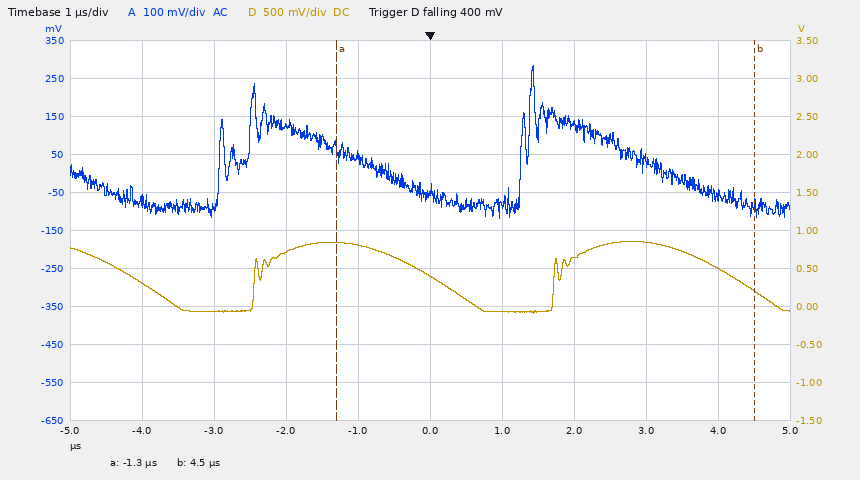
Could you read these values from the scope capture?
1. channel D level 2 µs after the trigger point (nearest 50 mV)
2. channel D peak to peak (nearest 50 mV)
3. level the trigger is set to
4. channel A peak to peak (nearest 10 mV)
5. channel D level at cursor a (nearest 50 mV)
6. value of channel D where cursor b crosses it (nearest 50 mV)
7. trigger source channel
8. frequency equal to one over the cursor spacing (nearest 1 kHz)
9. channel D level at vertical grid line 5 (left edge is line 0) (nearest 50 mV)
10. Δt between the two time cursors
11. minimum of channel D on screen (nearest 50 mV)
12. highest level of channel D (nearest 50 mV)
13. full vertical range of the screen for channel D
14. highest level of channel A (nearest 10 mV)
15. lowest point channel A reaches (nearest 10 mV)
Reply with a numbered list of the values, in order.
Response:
1. 650 mV
2. 950 mV
3. 400 mV
4. 400 mV
5. 850 mV
6. 200 mV
7. channel D
8. 172 kHz
9. 400 mV
10. 5.8 µs
11. -100 mV
12. 850 mV
13. 5 V
14. 280 mV
15. -120 mV
